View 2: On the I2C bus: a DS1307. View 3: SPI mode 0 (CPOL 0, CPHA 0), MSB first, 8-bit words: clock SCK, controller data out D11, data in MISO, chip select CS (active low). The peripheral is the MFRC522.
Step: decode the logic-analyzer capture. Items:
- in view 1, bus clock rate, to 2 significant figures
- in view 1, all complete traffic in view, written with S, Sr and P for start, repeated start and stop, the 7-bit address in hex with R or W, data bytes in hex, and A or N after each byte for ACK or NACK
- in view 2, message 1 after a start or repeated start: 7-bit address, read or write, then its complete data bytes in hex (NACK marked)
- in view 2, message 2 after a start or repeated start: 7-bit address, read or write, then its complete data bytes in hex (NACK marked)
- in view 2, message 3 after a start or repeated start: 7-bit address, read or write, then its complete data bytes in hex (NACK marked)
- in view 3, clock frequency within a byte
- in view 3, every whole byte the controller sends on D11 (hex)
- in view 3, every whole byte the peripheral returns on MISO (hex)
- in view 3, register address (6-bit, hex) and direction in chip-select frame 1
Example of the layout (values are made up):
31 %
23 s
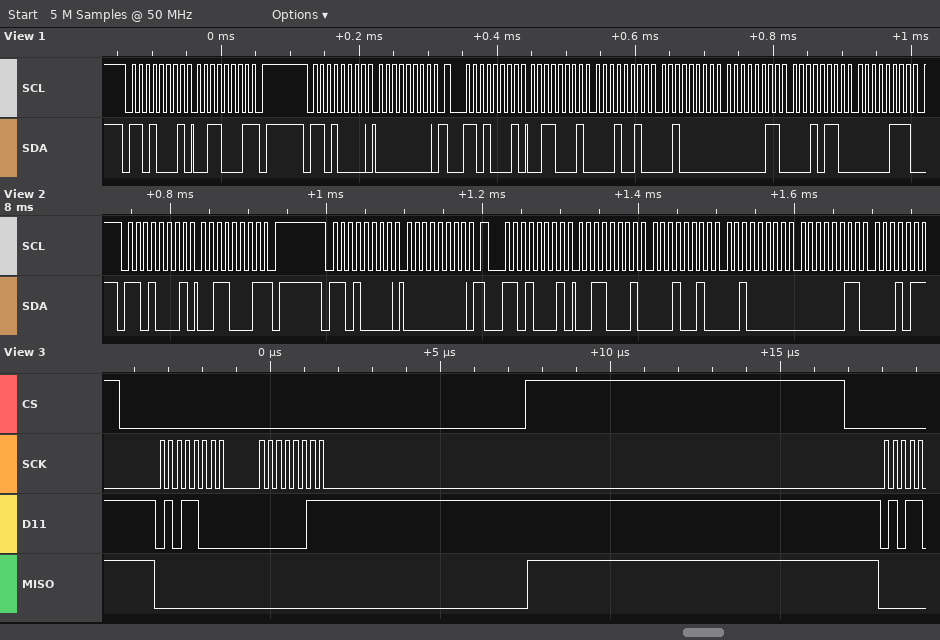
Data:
100 kHz
S 68R A 31 N P S 68W A 00 A Sr 68R A 31 A 12 A 20 A 03 A 16 A 07 A
0x68 read: 31 NACK
0x68 write: 00
0x68 read: 31 12 20 03
4 MHz
58 03
00 00
0x2C write
